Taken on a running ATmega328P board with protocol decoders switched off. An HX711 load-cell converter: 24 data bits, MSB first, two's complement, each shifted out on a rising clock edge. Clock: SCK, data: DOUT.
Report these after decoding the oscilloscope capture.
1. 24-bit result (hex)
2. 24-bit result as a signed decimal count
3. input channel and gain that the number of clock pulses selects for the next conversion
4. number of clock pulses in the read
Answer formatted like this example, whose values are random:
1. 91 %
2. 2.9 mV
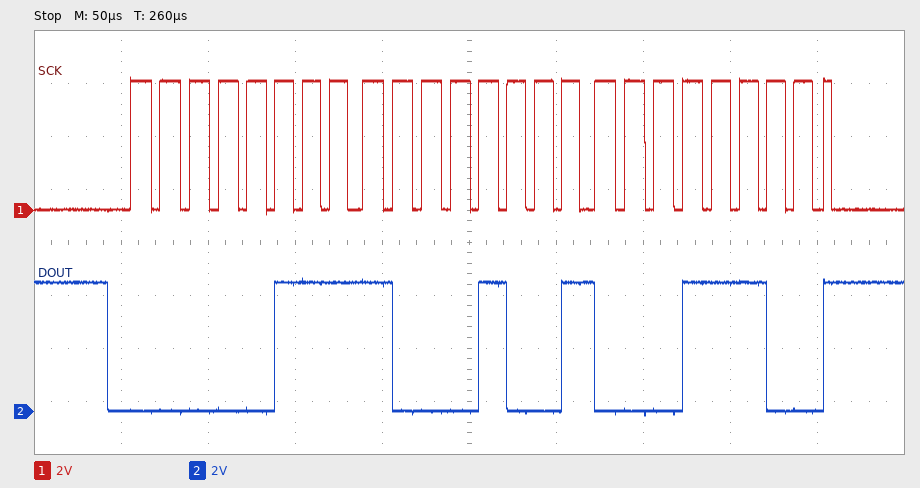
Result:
1. 0x07891C
2. 493852
3. channel A, gain 128
4. 25
